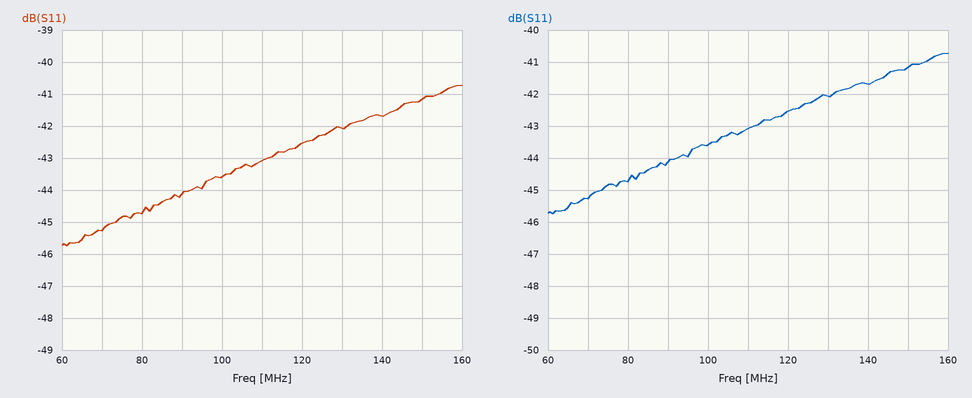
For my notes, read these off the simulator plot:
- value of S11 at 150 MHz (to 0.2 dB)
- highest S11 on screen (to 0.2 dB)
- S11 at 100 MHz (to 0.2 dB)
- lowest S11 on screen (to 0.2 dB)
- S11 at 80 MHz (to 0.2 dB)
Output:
-41.2 dB
-40.8 dB
-43.6 dB
-45.8 dB
-44.8 dB
